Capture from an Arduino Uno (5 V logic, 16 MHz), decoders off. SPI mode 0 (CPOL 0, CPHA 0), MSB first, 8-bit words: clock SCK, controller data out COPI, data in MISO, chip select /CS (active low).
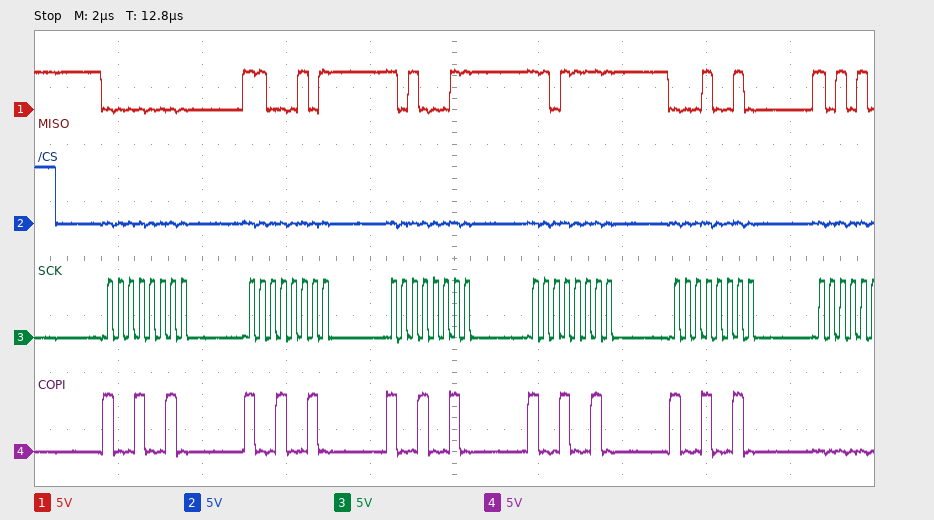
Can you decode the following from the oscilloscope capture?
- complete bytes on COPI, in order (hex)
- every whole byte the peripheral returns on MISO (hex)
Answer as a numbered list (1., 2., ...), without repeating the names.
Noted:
1. 92 92 92 92 92
2. 00 C5 A3 DF 12
